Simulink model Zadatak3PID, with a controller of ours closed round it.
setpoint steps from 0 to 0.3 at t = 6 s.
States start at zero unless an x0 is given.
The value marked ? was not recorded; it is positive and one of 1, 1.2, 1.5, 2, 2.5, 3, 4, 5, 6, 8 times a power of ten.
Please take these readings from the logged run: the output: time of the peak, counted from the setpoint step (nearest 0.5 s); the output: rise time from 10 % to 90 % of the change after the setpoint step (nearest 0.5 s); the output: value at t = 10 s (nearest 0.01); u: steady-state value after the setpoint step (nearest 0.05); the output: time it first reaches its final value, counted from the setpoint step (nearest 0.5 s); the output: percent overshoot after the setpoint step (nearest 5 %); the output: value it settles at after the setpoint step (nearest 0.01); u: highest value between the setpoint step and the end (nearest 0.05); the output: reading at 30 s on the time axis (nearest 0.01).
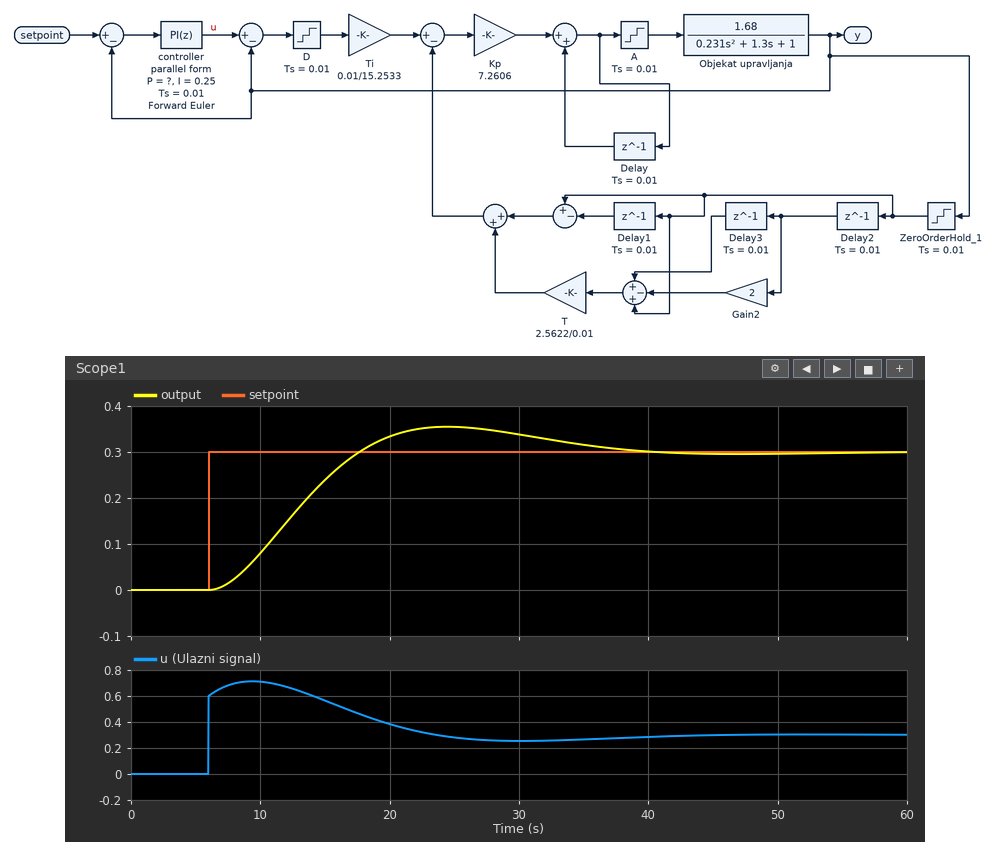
18.5 s
8.0 s
0.08
0.30
11.5 s
20 %
0.30
0.70
0.34
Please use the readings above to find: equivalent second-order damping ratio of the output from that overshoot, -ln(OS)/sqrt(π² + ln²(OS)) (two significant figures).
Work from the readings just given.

0.46
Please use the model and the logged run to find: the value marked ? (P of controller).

2
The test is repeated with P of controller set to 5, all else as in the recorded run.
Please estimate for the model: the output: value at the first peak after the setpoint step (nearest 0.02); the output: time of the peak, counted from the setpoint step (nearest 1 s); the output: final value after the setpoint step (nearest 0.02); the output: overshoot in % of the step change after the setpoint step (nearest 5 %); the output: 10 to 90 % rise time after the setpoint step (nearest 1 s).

0.34
10 s
0.30
10 %
5 s
